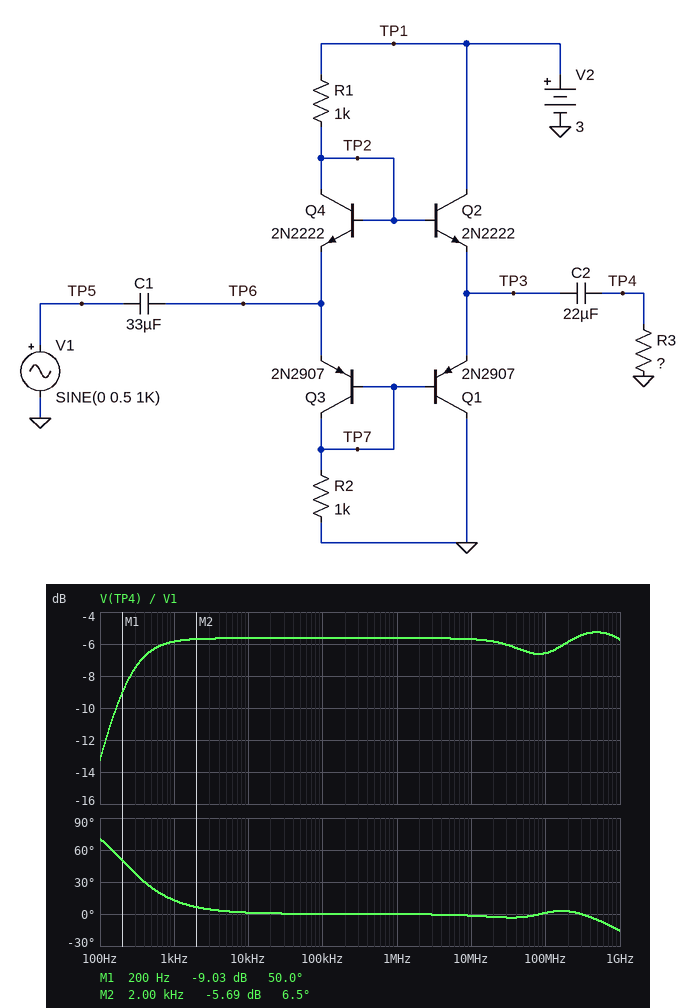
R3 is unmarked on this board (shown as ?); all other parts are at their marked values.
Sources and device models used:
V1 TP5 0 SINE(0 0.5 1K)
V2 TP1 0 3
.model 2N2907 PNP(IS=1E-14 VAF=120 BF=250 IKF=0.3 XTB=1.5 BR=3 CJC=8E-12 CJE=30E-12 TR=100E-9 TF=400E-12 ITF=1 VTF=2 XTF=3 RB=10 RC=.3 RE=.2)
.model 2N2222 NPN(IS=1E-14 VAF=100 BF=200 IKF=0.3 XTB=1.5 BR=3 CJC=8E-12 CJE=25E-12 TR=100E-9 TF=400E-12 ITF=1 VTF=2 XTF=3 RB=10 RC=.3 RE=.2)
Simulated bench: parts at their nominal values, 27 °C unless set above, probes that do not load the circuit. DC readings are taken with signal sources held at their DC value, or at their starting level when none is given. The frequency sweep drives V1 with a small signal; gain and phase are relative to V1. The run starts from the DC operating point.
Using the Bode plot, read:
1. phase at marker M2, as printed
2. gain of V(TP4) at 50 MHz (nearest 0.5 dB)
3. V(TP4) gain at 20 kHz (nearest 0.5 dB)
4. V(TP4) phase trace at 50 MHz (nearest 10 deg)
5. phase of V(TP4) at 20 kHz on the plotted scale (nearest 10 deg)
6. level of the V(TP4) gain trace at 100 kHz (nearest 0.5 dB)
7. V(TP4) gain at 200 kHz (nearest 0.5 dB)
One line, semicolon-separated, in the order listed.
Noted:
6.5 deg; -6.5 dB; -5.5 dB; 0 deg; 0 deg; -5.5 dB; -5.5 dB
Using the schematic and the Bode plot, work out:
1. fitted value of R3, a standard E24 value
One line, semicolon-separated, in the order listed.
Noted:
18 Ω
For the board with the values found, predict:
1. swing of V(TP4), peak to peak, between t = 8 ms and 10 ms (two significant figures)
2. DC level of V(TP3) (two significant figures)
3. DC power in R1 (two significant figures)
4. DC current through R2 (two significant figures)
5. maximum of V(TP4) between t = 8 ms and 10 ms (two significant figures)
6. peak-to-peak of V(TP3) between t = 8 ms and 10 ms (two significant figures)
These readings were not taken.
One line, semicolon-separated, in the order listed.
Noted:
720 mV; 1.5 V; 720 µW; 850 µA; 360 mV; 770 mV
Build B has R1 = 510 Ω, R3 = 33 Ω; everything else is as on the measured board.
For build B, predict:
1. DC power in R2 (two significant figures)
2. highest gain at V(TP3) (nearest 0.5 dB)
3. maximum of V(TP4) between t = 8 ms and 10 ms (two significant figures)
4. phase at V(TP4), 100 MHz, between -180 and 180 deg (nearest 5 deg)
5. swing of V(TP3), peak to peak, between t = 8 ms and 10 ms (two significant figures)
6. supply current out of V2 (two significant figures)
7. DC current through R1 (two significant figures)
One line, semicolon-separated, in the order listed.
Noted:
1.2 mW; -1.0 dB; 390 mV; -5 deg; 810 mV; 2.2 mA; 1.1 mA
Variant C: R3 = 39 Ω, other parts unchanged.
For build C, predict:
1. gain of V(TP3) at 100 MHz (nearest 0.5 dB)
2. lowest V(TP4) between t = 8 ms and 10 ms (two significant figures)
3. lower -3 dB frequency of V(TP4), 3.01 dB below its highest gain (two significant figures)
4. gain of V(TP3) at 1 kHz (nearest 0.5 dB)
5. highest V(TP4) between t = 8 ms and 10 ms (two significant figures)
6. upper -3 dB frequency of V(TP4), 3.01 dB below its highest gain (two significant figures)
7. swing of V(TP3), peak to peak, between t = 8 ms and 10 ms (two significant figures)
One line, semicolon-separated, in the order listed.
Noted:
-4.0 dB; -400 mV; 130 Hz; -3.0 dB; 400 mV; 1.9 GHz; 820 mV
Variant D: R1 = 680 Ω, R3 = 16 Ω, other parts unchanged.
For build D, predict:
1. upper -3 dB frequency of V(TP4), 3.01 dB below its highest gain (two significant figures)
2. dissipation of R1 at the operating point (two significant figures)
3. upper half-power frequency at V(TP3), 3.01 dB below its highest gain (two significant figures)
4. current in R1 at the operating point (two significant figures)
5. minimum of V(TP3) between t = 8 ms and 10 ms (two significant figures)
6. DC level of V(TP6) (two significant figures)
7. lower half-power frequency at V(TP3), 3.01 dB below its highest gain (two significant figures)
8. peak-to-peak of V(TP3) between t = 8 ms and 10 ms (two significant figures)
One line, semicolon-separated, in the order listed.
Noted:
3.3 GHz; 690 µW; 460 Hz; 1.0 mA; 1.3 V; 1.7 V; 11 Hz; 770 mV
